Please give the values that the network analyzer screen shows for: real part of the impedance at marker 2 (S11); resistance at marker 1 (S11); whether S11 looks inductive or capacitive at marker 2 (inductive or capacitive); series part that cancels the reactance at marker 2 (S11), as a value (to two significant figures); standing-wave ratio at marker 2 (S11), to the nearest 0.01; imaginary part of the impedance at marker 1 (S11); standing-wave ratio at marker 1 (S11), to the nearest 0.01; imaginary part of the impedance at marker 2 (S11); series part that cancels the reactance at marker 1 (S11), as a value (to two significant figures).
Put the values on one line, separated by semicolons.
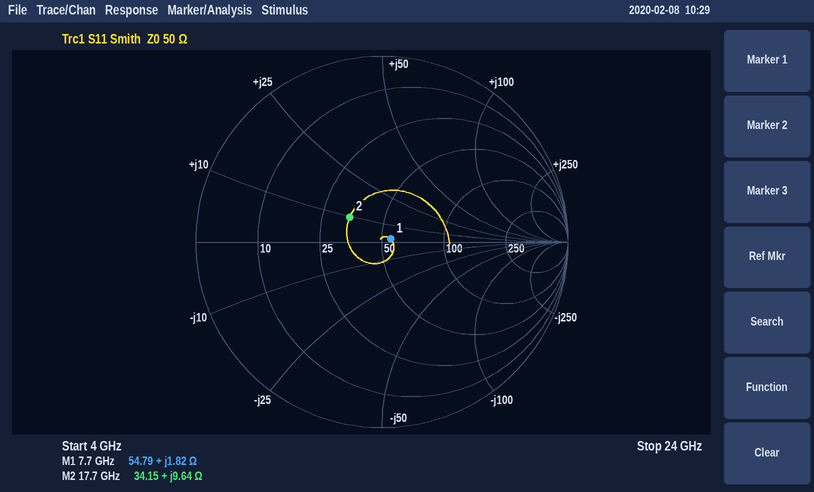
34.15 Ω; 54.79 Ω; inductive; 930 fF; 1.56; +1.82 Ω; 1.10; +9.64 Ω; 11 pF
